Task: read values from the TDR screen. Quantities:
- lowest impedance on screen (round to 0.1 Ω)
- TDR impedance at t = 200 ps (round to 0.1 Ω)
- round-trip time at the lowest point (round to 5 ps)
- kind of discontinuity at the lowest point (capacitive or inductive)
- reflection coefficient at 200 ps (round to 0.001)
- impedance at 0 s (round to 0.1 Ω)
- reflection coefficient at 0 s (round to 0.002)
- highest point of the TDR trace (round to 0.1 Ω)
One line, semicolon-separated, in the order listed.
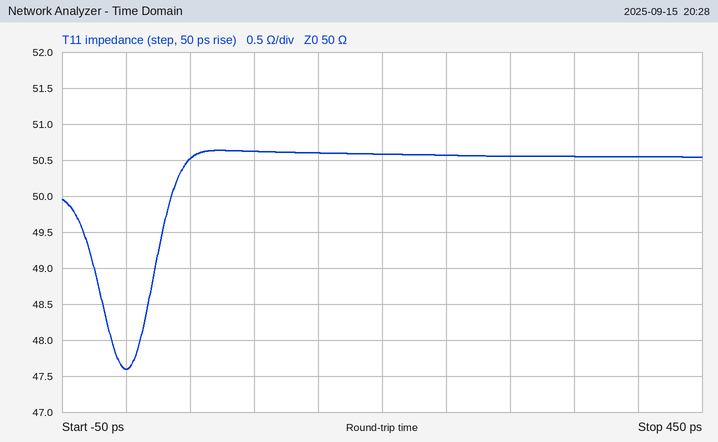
47.6 Ω; 50.6 Ω; 0 ps; capacitive; +0.006; 47.6 Ω; -0.024; 50.6 Ω
